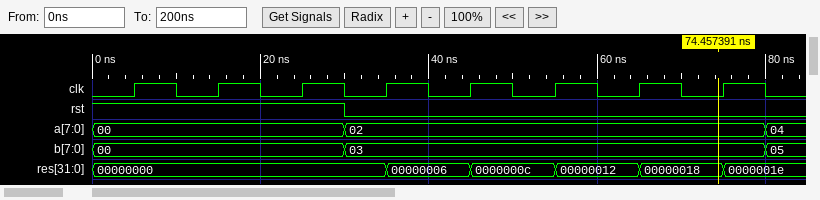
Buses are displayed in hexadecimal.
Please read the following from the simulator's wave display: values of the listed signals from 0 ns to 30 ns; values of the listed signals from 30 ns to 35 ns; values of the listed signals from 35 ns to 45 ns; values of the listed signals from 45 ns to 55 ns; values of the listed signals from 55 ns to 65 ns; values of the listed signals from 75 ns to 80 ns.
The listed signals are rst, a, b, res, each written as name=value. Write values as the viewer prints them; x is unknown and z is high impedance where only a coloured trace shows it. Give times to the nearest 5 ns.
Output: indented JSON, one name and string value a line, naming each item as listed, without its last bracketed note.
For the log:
{
  "values of the listed signals from 0 ns to 30 ns": "rst=1, a=00, b=00, res=00000000",
  "values of the listed signals from 30 ns to 35 ns": "rst=0, a=02, b=03, res=00000000",
  "values of the listed signals from 35 ns to 45 ns": "rst=0, a=02, b=03, res=00000006",
  "values of the listed signals from 45 ns to 55 ns": "rst=0, a=02, b=03, res=0000000c",
  "values of the listed signals from 55 ns to 65 ns": "rst=0, a=02, b=03, res=00000012",
  "values of the listed signals from 75 ns to 80 ns": "rst=0, a=02, b=03, res=0000001e"
}
